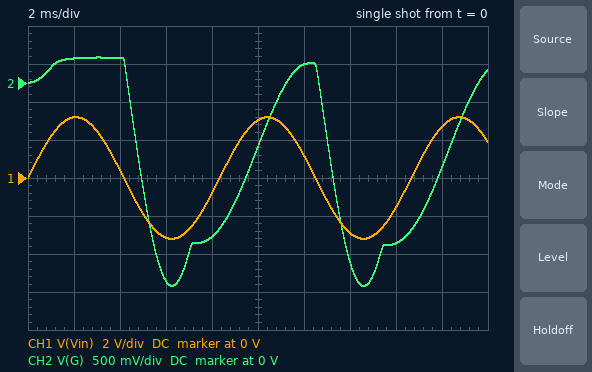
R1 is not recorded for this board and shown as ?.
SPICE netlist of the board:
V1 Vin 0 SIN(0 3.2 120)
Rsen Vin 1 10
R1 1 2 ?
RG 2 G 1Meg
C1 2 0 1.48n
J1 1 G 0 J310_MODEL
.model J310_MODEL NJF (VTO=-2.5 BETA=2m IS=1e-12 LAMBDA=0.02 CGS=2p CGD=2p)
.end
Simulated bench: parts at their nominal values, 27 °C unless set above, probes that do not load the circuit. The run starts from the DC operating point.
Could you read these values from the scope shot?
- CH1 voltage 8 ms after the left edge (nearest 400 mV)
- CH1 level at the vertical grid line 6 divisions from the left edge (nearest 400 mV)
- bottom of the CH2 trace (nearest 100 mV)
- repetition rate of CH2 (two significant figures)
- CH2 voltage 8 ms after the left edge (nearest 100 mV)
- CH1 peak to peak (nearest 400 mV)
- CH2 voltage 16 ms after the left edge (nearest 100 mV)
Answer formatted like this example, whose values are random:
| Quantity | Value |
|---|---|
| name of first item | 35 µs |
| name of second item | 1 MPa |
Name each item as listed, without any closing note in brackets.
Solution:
| Quantity | Value |
|---|---|
| CH1 voltage 8 ms after the left edge | -800 mV |
| CH1 level at the vertical grid line 6 divisions from the left edge | 1.2 V |
| bottom of the CH2 trace | -2.7 V |
| repetition rate of CH2 | 120 Hz |
| CH2 voltage 8 ms after the left edge | -2.0 V |
| CH1 peak to peak | 6.4 V |
| CH2 voltage 16 ms after the left edge | -2.1 V |
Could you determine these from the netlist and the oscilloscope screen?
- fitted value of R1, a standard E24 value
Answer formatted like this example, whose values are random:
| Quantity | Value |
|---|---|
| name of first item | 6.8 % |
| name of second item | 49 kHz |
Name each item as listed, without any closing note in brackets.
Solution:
| Quantity | Value |
|---|---|
| fitted value of R1, a standard E24 value | 3.3 MΩ |
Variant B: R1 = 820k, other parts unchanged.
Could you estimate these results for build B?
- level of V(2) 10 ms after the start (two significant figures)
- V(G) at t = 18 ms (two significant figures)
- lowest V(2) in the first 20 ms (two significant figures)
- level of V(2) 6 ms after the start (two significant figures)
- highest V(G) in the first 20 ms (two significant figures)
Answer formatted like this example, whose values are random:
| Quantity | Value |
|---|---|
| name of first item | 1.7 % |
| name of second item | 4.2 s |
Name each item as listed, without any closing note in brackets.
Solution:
| Quantity | Value |
|---|---|
| level of V(2) 10 ms after the start | 970 mV |
| V(G) at t = 18 ms | 320 mV |
| lowest V(2) in the first 20 ms | -2.6 V |
| level of V(2) 6 ms after the start | -2.0 V |
| highest V(G) in the first 20 ms | 360 mV |
